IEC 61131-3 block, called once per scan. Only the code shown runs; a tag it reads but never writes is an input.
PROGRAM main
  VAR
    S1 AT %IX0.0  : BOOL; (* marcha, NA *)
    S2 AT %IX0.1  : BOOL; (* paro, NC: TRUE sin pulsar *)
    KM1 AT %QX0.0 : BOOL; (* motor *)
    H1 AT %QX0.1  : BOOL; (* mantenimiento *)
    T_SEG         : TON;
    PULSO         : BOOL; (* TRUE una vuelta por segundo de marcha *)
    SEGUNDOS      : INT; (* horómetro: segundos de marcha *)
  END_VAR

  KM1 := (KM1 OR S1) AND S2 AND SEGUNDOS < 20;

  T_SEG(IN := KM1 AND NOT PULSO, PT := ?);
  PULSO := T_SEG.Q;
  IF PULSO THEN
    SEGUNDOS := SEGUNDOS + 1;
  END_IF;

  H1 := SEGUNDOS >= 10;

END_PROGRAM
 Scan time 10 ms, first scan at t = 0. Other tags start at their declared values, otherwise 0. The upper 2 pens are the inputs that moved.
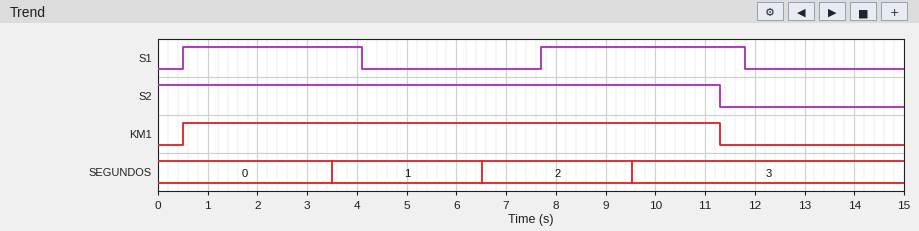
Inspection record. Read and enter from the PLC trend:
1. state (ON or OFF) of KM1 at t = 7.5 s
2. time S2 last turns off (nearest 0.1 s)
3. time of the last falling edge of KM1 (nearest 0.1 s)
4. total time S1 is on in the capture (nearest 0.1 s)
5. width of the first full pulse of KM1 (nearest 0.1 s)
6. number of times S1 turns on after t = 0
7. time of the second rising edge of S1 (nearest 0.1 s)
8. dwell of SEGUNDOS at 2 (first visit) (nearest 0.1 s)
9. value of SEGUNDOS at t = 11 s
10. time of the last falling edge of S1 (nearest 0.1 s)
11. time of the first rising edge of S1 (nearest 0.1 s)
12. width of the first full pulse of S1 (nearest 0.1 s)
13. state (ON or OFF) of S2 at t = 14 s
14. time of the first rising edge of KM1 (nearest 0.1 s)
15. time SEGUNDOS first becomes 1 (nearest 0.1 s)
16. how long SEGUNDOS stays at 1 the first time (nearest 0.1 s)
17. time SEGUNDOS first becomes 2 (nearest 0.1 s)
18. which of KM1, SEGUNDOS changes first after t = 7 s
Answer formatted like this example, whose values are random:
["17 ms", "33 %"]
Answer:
["ON", "11.3 s", "11.3 s", "7.7 s", "10.8 s", "2", "7.7 s", "3.0 s", "3", "11.8 s", "0.5 s", "3.6 s", "OFF", "0.5 s", "3.5 s", "3.0 s", "6.5 s", "SEGUNDOS"]
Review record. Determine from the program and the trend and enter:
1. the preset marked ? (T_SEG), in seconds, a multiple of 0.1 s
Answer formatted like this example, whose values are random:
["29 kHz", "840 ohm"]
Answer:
["3.0 s"]
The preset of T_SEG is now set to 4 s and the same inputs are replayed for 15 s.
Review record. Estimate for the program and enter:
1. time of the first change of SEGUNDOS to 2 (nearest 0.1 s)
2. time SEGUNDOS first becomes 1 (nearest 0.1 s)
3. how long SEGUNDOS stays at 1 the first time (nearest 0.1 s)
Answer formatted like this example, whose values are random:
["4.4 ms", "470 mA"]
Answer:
["8.5 s", "4.5 s", "4.0 s"]
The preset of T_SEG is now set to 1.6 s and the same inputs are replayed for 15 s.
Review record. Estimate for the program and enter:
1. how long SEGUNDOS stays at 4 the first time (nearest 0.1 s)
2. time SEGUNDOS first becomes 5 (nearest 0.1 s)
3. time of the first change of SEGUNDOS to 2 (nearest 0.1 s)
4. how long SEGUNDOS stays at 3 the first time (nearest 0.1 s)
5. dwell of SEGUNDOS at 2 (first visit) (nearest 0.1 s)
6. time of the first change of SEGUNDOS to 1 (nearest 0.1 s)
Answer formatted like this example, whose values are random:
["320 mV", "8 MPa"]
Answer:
["1.6 s", "8.6 s", "3.7 s", "1.6 s", "1.6 s", "2.1 s"]
